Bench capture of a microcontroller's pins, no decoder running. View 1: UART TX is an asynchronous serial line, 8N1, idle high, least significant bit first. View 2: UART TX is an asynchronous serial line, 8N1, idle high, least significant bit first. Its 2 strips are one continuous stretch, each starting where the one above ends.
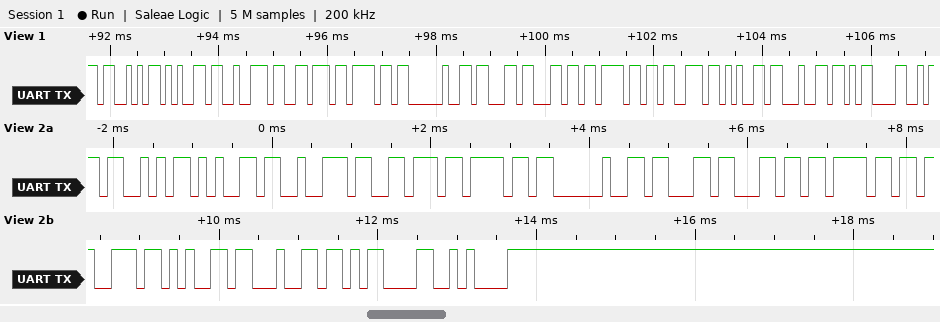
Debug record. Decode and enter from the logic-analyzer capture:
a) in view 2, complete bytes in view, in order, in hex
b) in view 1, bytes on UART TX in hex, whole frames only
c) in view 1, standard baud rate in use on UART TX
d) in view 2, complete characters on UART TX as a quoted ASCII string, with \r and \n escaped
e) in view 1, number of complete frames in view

53 65 72 76 6F 20 63 6C 6F 73 65 64 0D 0A
0x53 0x65 0x72 0x76 0x6F 0x20 0x63 0x6C 0x6F 0x73 0x65 0x64 0x0D
9600 baud
"Servo closed\r\n"
13
